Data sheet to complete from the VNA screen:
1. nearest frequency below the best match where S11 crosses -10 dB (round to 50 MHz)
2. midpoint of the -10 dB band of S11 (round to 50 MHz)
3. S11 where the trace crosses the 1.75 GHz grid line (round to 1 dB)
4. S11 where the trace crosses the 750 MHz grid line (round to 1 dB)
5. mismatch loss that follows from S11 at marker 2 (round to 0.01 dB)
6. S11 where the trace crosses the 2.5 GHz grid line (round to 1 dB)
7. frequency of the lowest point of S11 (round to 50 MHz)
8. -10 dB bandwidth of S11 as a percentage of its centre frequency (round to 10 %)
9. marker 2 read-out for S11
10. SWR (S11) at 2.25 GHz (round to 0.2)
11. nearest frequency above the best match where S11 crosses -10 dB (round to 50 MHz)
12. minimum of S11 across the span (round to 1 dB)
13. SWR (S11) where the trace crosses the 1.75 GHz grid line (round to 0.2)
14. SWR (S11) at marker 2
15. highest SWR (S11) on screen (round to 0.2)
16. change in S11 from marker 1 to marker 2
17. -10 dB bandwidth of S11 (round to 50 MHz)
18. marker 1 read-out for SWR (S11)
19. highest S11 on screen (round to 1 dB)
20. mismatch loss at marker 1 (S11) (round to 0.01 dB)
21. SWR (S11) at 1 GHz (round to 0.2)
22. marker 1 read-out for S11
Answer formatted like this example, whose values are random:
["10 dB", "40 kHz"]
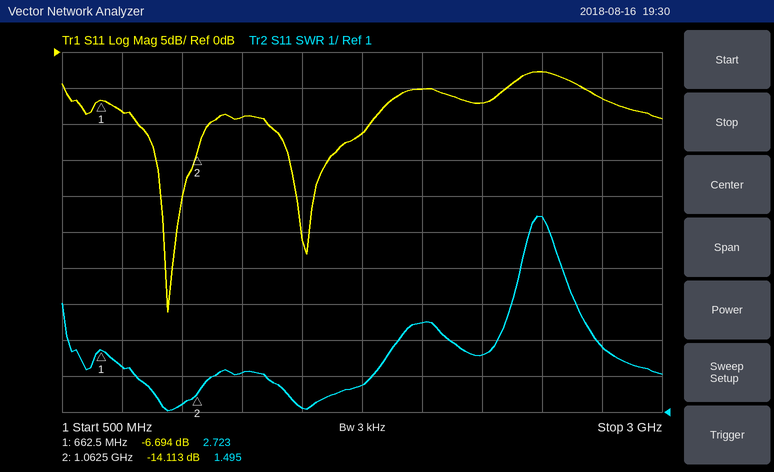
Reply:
["800 MHz", "950 MHz", "-11 dB", "-8 dB", "0.17 dB", "-3 dB", "950 MHz", "30 %", "-14.113 dB", "2.6", "1.10 GHz", "-36 dB", "1.8", "1.495", "6.4", "-7.419 dB", "300 MHz", "2.723", "-3 dB", "1.05 dB", "1.2", "-6.694 dB"]
